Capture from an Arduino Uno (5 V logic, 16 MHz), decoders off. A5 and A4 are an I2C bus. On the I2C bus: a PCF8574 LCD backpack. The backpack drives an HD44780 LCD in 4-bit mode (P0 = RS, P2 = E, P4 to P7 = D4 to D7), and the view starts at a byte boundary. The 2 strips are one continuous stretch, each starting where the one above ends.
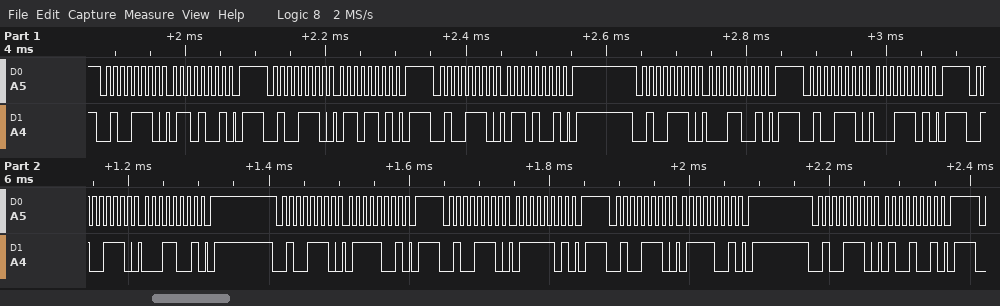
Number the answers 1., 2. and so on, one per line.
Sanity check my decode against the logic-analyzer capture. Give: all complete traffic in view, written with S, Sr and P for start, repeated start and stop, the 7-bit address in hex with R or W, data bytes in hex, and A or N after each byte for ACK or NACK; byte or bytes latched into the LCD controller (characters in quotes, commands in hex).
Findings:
1. S 27W A 69 A P S 27W A 6D A P S 27W A 69 A P S 27W A 19 A P S 27W A 1D A P S 27W A 19 A P S 27W A 79 A P S 27W A 7D A P S 27W A 79 A P S 27W A 49 A P
2. 'a'
